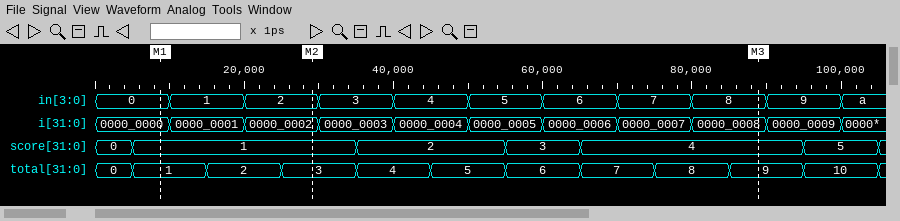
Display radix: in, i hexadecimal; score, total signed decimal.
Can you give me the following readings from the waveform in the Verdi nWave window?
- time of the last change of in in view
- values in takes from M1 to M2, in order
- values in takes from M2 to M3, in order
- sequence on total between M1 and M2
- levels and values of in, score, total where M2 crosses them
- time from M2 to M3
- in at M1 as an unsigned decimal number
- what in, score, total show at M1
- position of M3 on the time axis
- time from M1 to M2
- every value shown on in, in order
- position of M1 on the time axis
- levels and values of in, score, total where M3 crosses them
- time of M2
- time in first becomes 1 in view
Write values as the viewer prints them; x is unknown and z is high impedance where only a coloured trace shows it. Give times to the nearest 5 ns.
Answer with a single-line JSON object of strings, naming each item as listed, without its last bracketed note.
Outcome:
{"time of the last change of in in view": "100 ns", "values in takes from M1 to M2, in order": "0, 1, 2", "values in takes from M2 to M3, in order": "2, 3, 4, 5, 6, 7, 8", "sequence on total between M1 and M2": "1, 2, 3", "levels and values of in, score, total where M2 crosses them": "in=2, score=1, total=3", "time from M2 to M3": "60 ns", "in at M1 as an unsigned decimal number": "0", "what in, score, total show at M1": "in=0, score=1, total=1", "position of M3 on the time axis": "90 ns", "time from M1 to M2": "20 ns", "every value shown on in, in order": "0, 1, 2, 3, 4, 5, 6, 7, 8, 9, a", "position of M1 on the time axis": "10 ns", "levels and values of in, score, total where M3 crosses them": "in=8, score=4, total=9", "time of M2": "30 ns", "time in first becomes 1 in view": "10 ns"}
